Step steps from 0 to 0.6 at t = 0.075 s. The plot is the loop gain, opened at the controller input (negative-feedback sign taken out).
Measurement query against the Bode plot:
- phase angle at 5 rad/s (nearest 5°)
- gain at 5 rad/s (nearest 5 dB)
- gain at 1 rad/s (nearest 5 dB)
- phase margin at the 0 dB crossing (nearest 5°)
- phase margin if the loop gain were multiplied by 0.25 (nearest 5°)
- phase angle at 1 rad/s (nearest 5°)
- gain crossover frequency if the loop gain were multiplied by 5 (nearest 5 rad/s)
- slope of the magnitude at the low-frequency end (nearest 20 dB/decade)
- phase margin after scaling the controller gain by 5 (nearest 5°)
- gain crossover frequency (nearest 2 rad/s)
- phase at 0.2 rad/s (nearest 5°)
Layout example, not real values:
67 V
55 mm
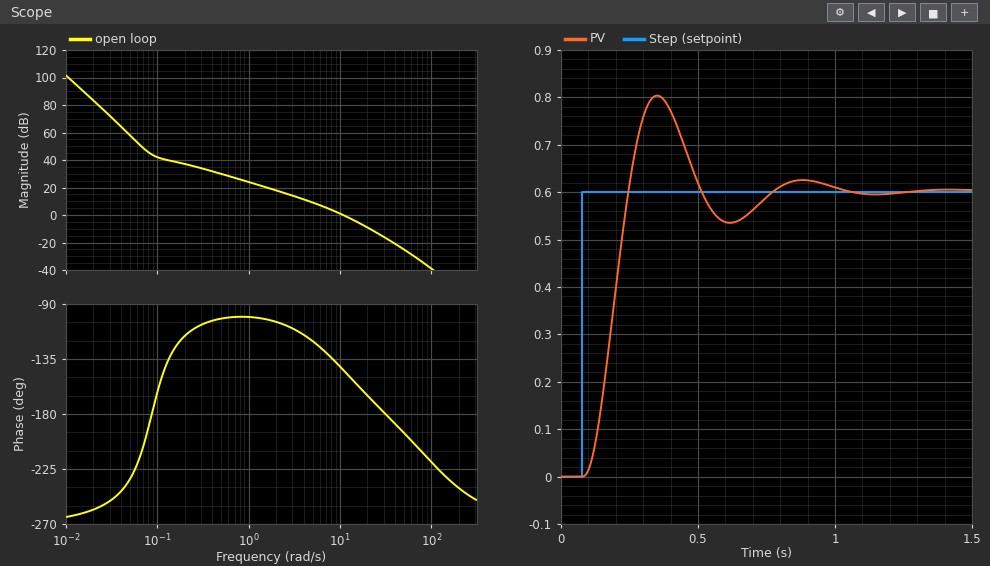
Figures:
-120°
10 dB
25 dB
35°
65°
-100°
25 rad/s
-60 dB/decade
5°
10 rad/s
-115°
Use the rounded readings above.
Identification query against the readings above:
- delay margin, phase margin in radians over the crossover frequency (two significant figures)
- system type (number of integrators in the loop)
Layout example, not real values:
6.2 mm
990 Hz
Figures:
0.061 s
3
